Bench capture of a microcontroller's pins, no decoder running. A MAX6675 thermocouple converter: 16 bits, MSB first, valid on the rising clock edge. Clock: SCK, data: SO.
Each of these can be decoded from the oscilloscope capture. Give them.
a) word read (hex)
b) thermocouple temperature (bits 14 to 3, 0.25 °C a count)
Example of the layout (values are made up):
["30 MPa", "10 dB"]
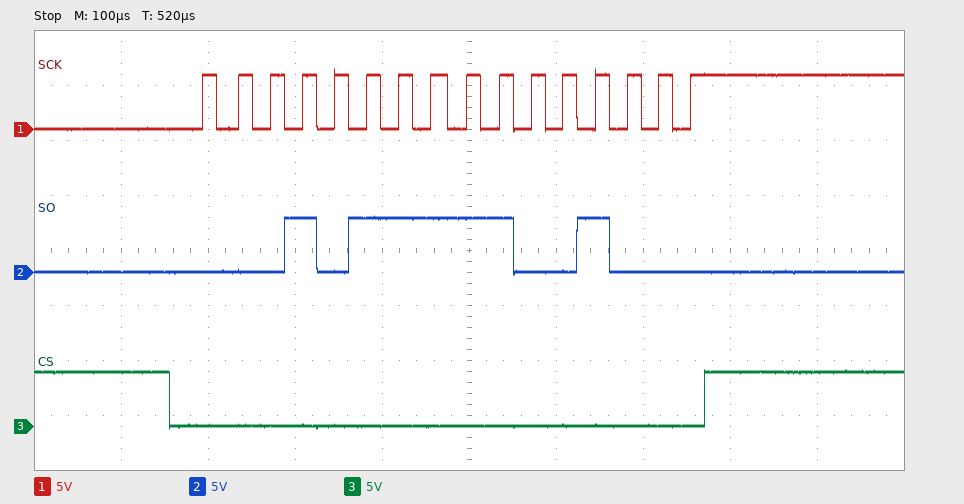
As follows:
["0x17C8", "190.25 °C"]
